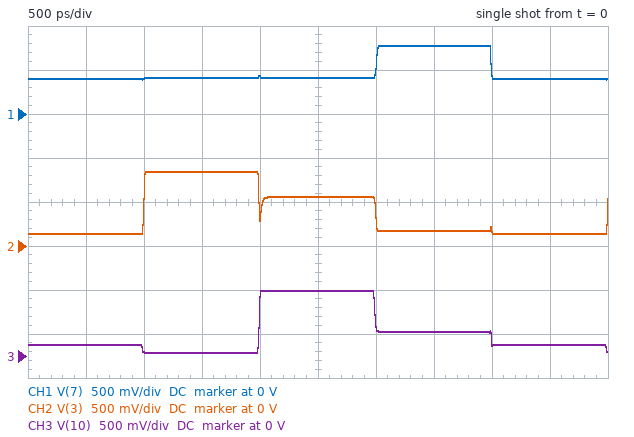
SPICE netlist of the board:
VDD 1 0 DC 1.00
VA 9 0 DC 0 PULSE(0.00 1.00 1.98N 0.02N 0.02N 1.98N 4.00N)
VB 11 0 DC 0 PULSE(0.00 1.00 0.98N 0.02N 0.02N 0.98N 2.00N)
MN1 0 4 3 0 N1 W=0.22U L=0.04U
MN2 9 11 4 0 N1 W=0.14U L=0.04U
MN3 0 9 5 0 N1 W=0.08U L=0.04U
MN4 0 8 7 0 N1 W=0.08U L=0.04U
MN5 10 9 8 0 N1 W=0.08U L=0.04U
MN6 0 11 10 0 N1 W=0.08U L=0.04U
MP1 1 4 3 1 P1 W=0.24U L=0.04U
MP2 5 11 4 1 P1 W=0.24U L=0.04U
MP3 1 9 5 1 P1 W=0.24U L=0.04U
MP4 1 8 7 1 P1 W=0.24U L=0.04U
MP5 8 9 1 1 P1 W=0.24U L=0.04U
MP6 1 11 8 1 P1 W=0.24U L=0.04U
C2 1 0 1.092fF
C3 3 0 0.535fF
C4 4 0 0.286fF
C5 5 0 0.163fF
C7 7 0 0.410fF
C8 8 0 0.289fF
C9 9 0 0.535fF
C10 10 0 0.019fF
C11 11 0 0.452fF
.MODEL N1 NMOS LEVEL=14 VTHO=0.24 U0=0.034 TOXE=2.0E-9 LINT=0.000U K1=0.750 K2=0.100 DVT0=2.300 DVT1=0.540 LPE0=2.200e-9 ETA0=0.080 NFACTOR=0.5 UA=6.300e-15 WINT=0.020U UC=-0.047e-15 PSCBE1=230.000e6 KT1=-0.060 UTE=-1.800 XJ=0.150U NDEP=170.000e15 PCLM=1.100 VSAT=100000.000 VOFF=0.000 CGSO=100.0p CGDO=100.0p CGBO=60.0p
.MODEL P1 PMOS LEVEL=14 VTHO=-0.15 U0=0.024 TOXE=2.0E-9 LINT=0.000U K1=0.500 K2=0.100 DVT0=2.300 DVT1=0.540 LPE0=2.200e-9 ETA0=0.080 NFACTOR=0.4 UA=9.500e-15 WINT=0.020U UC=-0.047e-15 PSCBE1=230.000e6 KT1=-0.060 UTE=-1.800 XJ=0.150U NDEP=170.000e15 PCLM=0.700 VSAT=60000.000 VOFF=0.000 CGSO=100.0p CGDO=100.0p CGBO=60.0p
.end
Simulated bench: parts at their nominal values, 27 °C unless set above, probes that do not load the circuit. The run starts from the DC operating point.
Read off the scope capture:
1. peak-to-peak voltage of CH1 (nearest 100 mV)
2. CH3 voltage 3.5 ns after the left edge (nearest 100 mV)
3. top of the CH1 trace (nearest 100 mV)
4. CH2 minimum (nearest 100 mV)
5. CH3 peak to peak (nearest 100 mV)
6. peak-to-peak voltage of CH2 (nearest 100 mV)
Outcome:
400 mV
300 mV
800 mV
100 mV
700 mV
700 mV
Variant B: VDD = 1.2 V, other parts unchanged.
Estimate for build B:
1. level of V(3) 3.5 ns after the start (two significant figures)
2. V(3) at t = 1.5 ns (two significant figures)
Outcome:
260 mV
890 mV
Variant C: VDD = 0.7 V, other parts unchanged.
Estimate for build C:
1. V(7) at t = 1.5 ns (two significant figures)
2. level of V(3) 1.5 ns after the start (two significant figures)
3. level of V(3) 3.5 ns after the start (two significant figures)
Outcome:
310 mV
660 mV
20 mV
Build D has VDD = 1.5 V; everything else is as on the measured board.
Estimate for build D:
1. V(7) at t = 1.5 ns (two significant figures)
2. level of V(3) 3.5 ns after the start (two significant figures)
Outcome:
590 mV
300 mV
